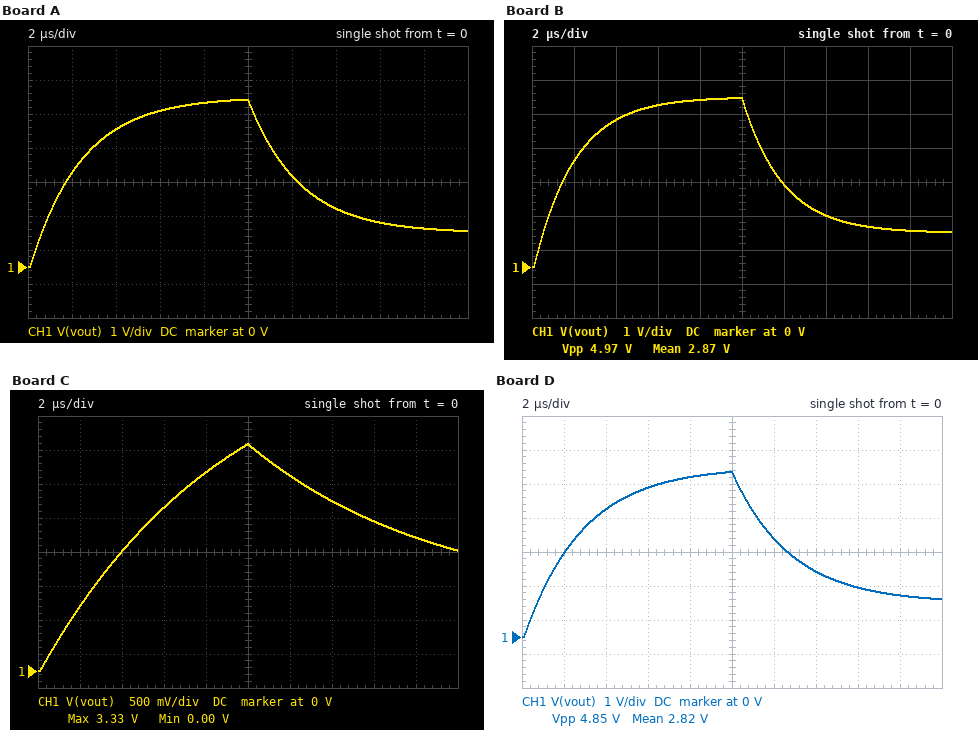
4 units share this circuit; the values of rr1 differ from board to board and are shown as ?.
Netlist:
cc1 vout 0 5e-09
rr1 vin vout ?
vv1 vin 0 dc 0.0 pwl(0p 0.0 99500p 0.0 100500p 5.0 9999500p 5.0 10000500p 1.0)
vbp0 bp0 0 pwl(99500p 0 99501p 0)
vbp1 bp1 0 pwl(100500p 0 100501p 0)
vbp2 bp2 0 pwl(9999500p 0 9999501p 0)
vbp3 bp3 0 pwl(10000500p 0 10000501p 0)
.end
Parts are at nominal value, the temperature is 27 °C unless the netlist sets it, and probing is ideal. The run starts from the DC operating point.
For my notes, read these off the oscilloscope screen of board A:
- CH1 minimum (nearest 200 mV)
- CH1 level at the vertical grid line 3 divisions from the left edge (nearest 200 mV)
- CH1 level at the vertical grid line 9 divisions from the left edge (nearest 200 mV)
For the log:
0 V
4.6 V
1.2 V
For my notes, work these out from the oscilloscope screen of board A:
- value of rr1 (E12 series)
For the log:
470 Ω
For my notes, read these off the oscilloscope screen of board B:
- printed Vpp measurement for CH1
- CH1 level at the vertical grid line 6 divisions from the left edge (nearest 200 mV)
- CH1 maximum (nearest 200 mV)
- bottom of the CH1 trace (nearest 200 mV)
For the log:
4.97 V
2.4 V
5.0 V
0 V
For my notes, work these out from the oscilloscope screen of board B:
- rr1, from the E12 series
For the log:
390 Ω
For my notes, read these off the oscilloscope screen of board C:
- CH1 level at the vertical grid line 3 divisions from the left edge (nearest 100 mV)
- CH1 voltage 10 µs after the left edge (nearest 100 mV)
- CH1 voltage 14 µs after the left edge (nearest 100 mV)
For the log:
2.4 V
3.3 V
2.5 V
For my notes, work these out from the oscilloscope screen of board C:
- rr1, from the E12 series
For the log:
1.8 kΩ
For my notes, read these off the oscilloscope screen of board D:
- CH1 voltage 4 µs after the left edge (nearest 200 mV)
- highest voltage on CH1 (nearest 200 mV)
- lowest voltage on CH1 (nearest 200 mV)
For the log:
3.8 V
4.8 V
0 V
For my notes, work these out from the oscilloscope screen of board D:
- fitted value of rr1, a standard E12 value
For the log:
560 Ω
